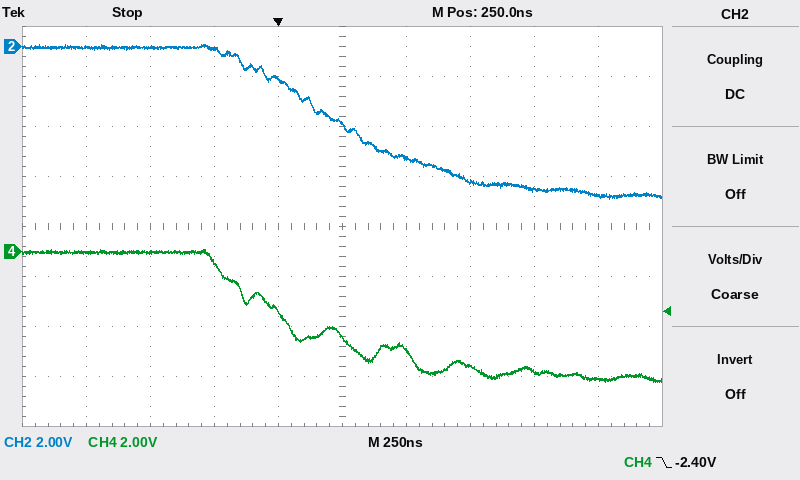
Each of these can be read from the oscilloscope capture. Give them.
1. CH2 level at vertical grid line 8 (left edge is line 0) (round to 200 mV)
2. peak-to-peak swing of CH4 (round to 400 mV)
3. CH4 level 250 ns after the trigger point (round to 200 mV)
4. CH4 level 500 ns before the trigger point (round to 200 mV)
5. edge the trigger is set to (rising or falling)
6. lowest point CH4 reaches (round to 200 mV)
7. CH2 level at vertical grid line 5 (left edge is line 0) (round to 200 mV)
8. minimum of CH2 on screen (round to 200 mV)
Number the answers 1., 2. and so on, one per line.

1. -5.8 V
2. 5.2 V
3. -3.4 V
4. 0.0 V
5. falling
6. -5.2 V
7. -3.2 V
8. -6.2 V
